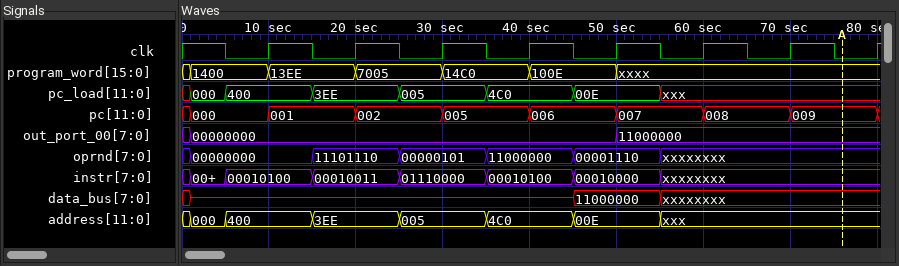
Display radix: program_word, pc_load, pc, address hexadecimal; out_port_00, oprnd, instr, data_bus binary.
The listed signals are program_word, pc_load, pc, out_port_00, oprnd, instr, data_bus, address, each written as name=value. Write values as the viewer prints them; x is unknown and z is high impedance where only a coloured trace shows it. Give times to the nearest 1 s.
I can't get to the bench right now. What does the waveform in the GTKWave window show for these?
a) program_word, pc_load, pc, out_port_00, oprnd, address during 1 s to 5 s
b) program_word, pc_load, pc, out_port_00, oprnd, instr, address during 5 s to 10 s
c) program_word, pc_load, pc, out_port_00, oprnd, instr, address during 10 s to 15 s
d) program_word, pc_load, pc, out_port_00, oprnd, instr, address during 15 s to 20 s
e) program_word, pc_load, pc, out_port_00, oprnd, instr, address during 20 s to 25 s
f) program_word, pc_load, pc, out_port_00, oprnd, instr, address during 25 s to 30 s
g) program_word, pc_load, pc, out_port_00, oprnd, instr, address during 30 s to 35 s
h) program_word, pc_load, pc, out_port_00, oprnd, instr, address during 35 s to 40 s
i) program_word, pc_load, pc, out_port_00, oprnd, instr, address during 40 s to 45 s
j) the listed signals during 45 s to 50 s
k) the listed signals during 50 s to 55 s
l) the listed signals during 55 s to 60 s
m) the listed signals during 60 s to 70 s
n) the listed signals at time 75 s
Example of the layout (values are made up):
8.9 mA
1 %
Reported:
program_word=1400, pc_load=000, pc=000, out_port_00=00000000, oprnd=00000000, address=000
program_word=1400, pc_load=400, pc=000, out_port_00=00000000, oprnd=00000000, instr=00010100, address=400
program_word=13EE, pc_load=400, pc=001, out_port_00=00000000, oprnd=00000000, instr=00010100, address=400
program_word=13EE, pc_load=3EE, pc=001, out_port_00=00000000, oprnd=11101110, instr=00010011, address=3EE
program_word=7005, pc_load=3EE, pc=002, out_port_00=00000000, oprnd=11101110, instr=00010011, address=3EE
program_word=7005, pc_load=005, pc=002, out_port_00=00000000, oprnd=00000101, instr=01110000, address=005
program_word=14C0, pc_load=005, pc=005, out_port_00=00000000, oprnd=00000101, instr=01110000, address=005
program_word=14C0, pc_load=4C0, pc=005, out_port_00=00000000, oprnd=11000000, instr=00010100, address=4C0
program_word=100E, pc_load=4C0, pc=006, out_port_00=00000000, oprnd=11000000, instr=00010100, address=4C0
program_word=100E, pc_load=00E, pc=006, out_port_00=00000000, oprnd=00001110, instr=00010000, data_bus=11000000, address=00E
program_word=xxxx, pc_load=00E, pc=007, out_port_00=11000000, oprnd=00001110, instr=00010000, data_bus=11000000, address=00E
program_word=xxxx, pc_load=xxx, pc=007, out_port_00=11000000, oprnd=xxxxxxxx, instr=xxxxxxxx, data_bus=xxxxxxxx, address=xxx
program_word=xxxx, pc_load=xxx, pc=008, out_port_00=11000000, oprnd=xxxxxxxx, instr=xxxxxxxx, data_bus=xxxxxxxx, address=xxx
program_word=xxxx, pc_load=xxx, pc=009, out_port_00=11000000, oprnd=xxxxxxxx, instr=xxxxxxxx, data_bus=xxxxxxxx, address=xxx
